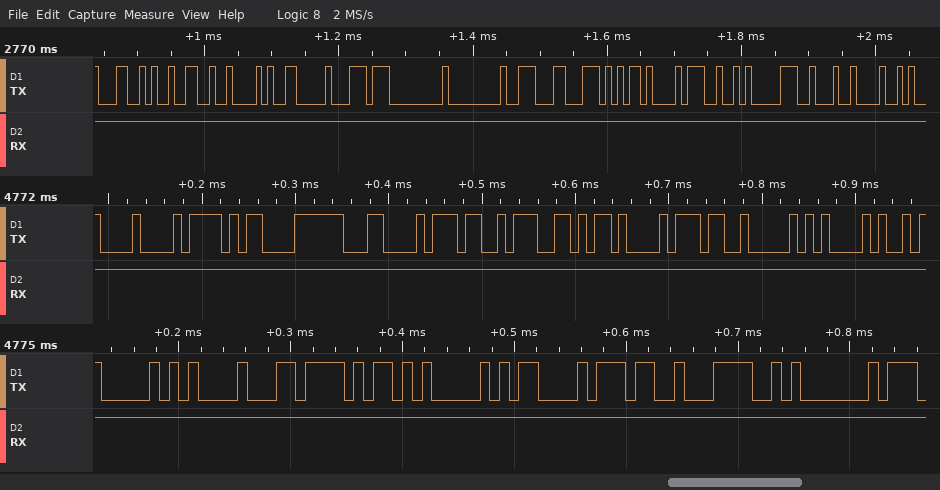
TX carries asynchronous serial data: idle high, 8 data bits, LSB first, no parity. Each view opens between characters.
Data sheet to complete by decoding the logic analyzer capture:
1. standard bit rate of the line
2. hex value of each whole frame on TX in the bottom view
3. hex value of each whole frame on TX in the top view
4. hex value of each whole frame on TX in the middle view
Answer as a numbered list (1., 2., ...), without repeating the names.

1. 115200 baud
2. 50, 88, AF, 05, 0D, 37, 3C, 01
3. 4C, 32, 42, 06, DC, 00, 00, 8E, 5C, 0B, 27, C1, 22, 48
4. 08, AF, F8, 0C, 37, 67, 0B, 37, 50, 28
